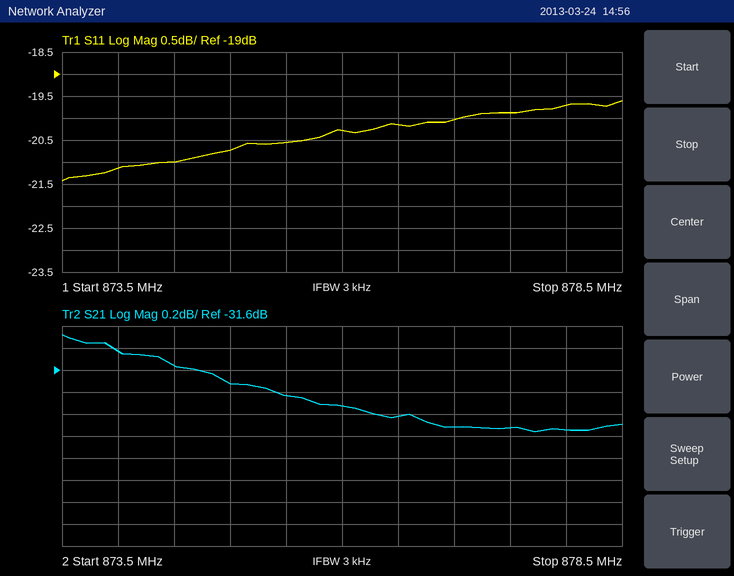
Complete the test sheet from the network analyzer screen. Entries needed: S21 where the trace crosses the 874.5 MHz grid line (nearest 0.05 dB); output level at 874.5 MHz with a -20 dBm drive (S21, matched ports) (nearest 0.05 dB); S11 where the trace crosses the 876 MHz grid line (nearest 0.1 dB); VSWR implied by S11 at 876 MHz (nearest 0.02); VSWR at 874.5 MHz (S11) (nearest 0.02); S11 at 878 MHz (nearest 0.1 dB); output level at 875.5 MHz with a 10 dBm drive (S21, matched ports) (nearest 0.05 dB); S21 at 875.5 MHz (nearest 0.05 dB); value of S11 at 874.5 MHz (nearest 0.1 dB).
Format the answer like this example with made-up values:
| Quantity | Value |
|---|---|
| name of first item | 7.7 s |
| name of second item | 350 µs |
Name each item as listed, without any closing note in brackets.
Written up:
| Quantity | Value |
|---|---|
| S21 where the trace crosses the 874.5 MHz grid line | -31.55 dB |
| output level at 874.5 MHz with a -20 dBm drive (S21, matched ports) | -51.55 dBm |
| S11 where the trace crosses the 876 MHz grid line | -20.3 dB |
| VSWR implied by S11 at 876 MHz | 1.22 |
| VSWR at 874.5 MHz (S11) | 1.20 |
| S11 at 878 MHz | -19.7 dB |
| output level at 875.5 MHz with a 10 dBm drive (S21, matched ports) | -21.85 dBm |
| S21 at 875.5 MHz | -31.85 dB |
| value of S11 at 874.5 MHz | -21.0 dB |
